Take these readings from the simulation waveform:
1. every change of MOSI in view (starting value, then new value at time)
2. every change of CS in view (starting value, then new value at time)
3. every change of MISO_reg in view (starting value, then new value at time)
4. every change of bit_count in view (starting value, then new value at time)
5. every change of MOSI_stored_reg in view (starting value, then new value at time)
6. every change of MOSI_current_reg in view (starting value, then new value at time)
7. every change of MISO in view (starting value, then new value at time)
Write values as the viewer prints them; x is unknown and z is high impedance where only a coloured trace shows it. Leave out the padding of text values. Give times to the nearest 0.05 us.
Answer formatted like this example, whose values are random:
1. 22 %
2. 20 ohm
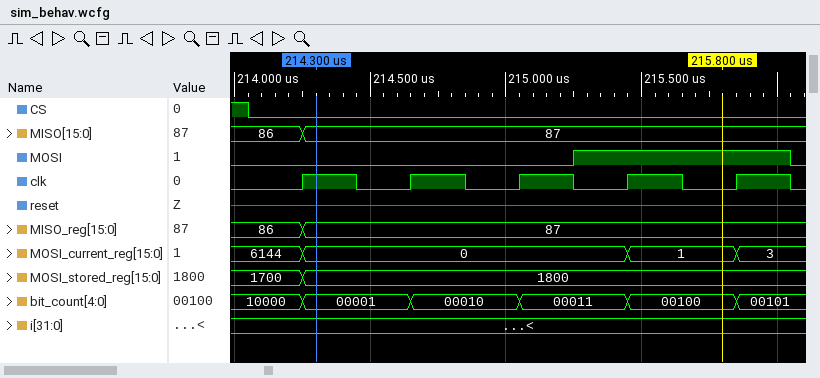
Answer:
1. 0, 1 at 215.25 us, 0 at 216.05 us
2. 1, 0 at 214.05 us
3. 86, 87 at 214.25 us
4. 10000, 00001 at 214.25 us, 00010 at 214.65 us, 00011 at 215.05 us, 00100 at 215.45 us, 00101 at 215.85 us
5. 1700, 1800 at 214.25 us
6. 6144, 0 at 214.25 us, 1 at 215.45 us, 3 at 215.85 us
7. 86, 87 at 214.25 us
